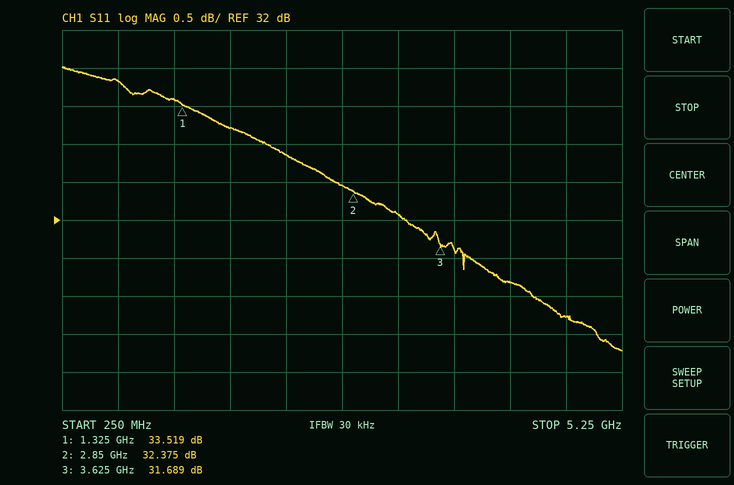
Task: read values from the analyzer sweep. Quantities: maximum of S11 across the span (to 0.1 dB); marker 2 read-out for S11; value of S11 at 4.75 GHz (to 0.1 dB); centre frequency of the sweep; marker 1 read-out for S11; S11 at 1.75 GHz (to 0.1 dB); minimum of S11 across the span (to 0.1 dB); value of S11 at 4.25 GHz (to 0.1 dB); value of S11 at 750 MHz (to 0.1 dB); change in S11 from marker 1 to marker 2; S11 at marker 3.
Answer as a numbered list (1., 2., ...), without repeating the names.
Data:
1. 34.0 dB
2. 32.375 dB
3. 30.7 dB
4. 2.75 GHz
5. 33.519 dB
6. 33.2 dB
7. 30.3 dB
8. 31.2 dB
9. 33.8 dB
10. -1.144 dB
11. 31.689 dB
